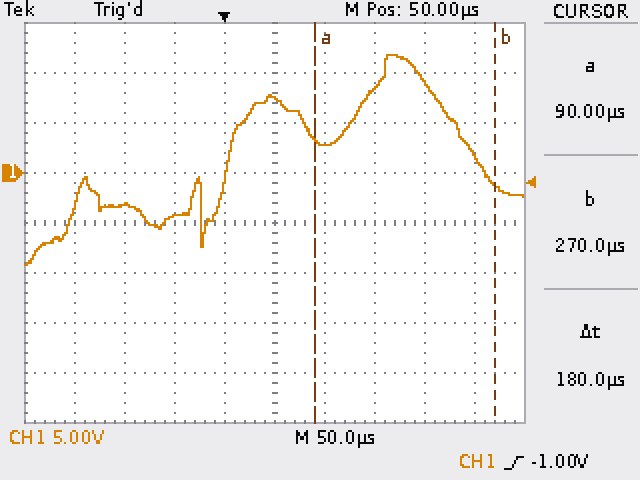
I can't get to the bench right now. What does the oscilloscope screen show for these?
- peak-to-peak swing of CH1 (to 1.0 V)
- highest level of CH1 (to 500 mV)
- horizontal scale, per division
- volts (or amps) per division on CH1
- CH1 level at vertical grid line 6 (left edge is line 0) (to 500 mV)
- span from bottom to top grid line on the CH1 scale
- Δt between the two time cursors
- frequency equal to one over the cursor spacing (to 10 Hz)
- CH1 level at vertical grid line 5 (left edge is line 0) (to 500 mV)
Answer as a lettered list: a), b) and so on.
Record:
a) 21.0 V
b) 12.0 V
c) 50 µs
d) 5 V
e) 3.0 V
f) 40 V
g) 180 µs
h) 5.56 kHz
i) 7.5 V
